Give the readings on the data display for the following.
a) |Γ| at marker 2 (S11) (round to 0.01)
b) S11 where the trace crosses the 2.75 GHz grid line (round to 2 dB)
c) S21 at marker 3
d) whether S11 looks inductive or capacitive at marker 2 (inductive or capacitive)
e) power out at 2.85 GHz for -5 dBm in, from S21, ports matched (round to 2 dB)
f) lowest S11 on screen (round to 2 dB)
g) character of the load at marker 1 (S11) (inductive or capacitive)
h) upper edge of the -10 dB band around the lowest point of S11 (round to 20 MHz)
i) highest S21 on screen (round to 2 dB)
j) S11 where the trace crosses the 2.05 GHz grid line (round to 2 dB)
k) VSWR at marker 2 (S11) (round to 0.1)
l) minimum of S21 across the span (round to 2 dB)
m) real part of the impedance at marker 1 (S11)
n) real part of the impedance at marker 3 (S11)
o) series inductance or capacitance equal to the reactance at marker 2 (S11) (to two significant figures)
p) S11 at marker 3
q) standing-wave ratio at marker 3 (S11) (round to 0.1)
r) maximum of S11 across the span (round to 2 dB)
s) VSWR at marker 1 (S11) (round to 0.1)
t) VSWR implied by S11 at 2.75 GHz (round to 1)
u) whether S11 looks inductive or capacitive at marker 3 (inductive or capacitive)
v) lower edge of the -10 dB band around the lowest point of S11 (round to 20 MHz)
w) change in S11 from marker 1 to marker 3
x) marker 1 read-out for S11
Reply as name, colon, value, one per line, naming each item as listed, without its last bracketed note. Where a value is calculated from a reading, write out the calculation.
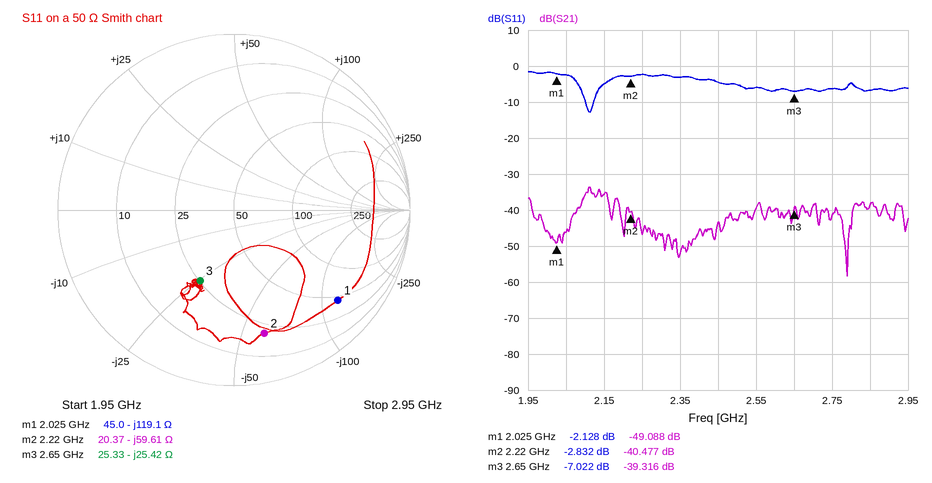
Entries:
|Γ| at marker 2 (S11): 0.72
S11 where the trace crosses the 2.75 GHz grid line: -6 dB
S21 at marker 3: -39.316 dB
whether S11 looks inductive or capacitive at marker 2: capacitive
power out at 2.85 GHz for -5 dBm in, from S21, ports matched: -5 dBm + (-38 dB) = -44 dBm
lowest S11 on screen: -12 dB
character of the load at marker 1 (S11): capacitive
upper edge of the -10 dB band around the lowest point of S11: 2.12 GHz
highest S21 on screen: -34 dB
S11 where the trace crosses the 2.05 GHz grid line: -2 dB
VSWR at marker 2 (S11): (1 + 0.7218)/(1 − 0.7218) ≈ 6.2
minimum of S21 across the span: -58 dB
real part of the impedance at marker 1: 45.0 Ω
real part of the impedance at marker 3: 25.33 Ω
series inductance or capacitance equal to the reactance at marker 2 (S11): C = 1/(2π × 2.22 GHz × 59.61 Ω) ≈ 1.2 pF
S11 at marker 3: -7.022 dB
standing-wave ratio at marker 3 (S11): 2.6
maximum of S11 across the span: -2 dB
VSWR at marker 1 (S11): 8.2
VSWR implied by S11 at 2.75 GHz: |Γ| = 10^(-6/20) = 0.5012; VSWR = (1 + 0.5012)/(1 − 0.5012) ≈ 3
whether S11 looks inductive or capacitive at marker 3: capacitive
lower edge of the -10 dB band around the lowest point of S11: 2.10 GHz
change in S11 from marker 1 to marker 3: -7.022 − (-2.128) = -4.894 dB
marker 1 read-out for S11: -2.128 dB
